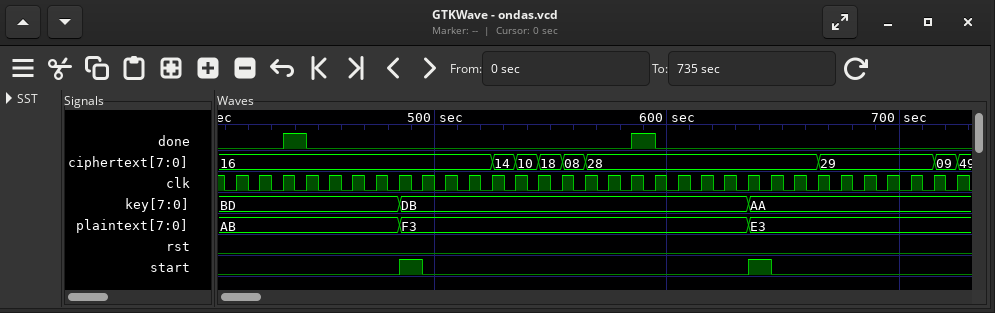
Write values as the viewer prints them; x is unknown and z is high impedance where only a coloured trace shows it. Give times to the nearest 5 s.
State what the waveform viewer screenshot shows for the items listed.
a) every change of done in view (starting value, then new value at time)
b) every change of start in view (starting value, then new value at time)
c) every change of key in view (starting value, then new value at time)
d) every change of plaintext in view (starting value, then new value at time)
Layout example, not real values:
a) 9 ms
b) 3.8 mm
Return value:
a) 0, 1 at 435 s, 0 at 445 s, 1 at 585 s, 0 at 595 s
b) 0, 1 at 485 s, 0 at 495 s, 1 at 635 s, 0 at 645 s
c) BD, DB at 485 s, AA at 635 s
d) AB, F3 at 485 s, E3 at 635 s
